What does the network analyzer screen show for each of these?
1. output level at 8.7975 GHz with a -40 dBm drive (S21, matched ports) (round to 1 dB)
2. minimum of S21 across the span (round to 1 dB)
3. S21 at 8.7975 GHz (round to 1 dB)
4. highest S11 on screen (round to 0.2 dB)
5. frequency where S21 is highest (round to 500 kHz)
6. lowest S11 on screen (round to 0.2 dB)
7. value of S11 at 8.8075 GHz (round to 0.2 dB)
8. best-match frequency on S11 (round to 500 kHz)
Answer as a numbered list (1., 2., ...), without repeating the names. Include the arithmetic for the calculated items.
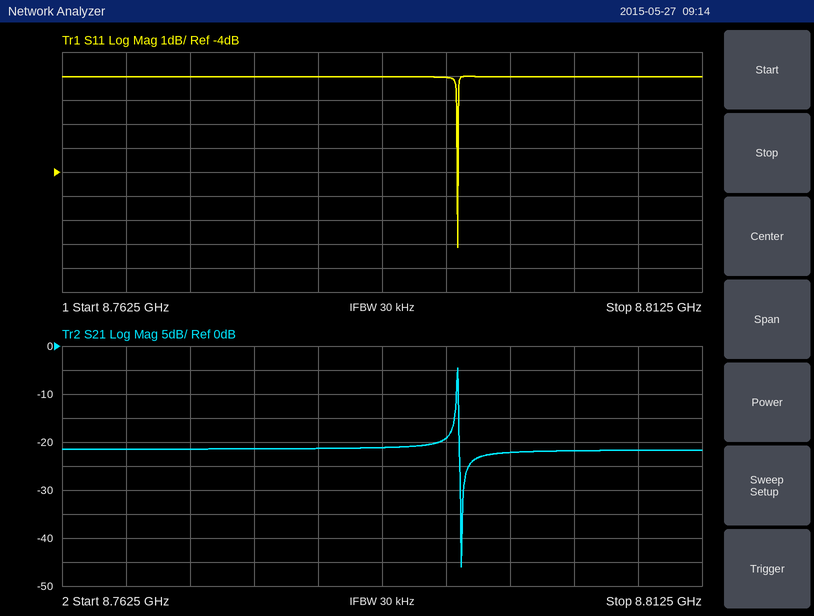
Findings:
1. -40 dBm + (-22 dB) = -62 dBm
2. -46 dB
3. -22 dB
4. 0.0 dB
5. 8.7935 GHz
6. -7.2 dB
7. 0.0 dB
8. 8.7935 GHz
